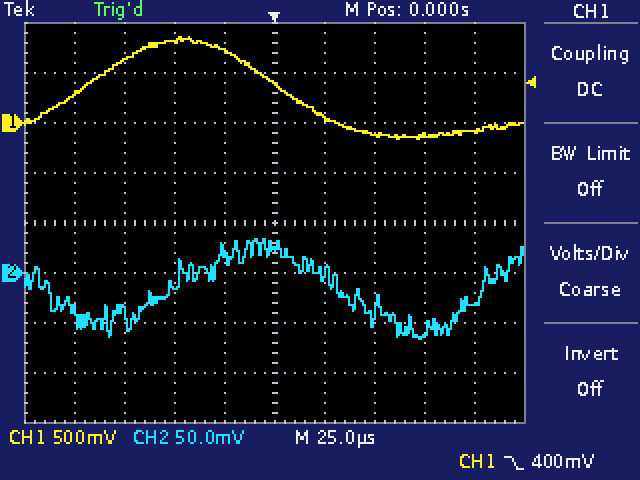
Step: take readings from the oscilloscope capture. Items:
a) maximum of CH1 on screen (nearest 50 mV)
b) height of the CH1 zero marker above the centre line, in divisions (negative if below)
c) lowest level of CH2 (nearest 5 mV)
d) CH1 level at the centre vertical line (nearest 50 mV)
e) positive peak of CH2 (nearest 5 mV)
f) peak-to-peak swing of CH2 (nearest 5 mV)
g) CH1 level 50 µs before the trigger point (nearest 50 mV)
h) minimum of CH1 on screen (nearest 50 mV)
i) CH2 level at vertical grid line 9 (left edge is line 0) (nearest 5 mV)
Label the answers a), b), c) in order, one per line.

a) 850 mV
b) +2.0 div
c) -65 mV
d) 400 mV
e) 35 mV
f) 100 mV
g) 800 mV
h) -150 mV
i) -30 mV
